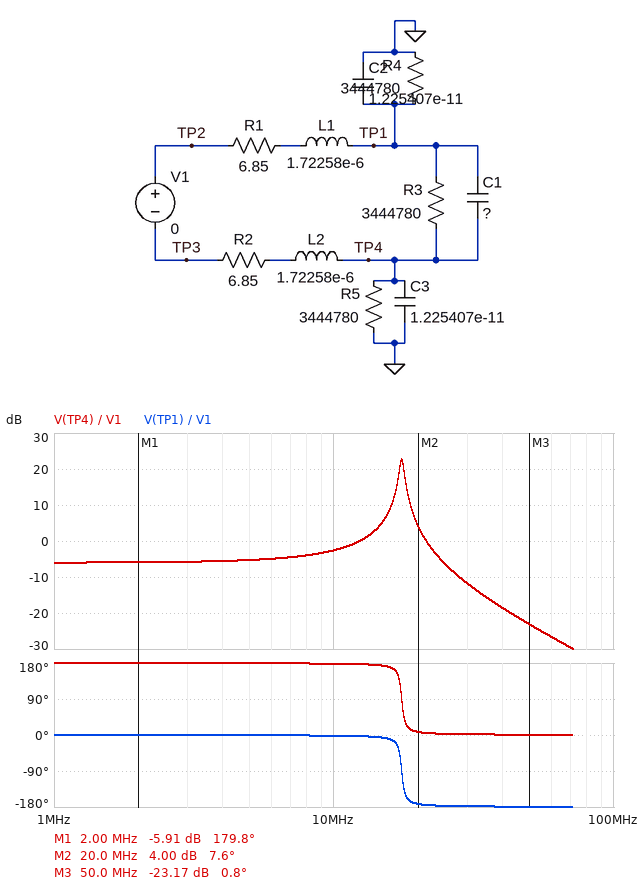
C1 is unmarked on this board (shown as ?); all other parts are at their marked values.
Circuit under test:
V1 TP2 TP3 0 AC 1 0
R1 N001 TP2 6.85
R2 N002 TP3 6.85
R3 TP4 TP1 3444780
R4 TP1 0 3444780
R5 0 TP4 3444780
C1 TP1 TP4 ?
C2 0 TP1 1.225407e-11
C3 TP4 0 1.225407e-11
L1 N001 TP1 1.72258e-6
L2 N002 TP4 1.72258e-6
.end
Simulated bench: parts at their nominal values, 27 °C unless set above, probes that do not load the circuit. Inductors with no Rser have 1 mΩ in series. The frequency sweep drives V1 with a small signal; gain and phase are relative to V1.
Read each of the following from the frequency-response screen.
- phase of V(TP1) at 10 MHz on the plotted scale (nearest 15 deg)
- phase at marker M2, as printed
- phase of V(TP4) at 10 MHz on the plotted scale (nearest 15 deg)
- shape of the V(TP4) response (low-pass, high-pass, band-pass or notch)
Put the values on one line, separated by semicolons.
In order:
0 deg; 7.6 deg; 180 deg; low-pass
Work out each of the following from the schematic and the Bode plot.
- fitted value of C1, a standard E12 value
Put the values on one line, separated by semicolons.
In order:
18 pF
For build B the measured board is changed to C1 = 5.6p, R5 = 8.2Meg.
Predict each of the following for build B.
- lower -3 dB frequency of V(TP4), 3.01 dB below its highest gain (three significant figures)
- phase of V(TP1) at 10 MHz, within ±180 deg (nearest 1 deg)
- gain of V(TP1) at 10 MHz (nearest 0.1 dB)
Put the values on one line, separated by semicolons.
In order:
24.7 MHz; -1 deg; -4.5 dB
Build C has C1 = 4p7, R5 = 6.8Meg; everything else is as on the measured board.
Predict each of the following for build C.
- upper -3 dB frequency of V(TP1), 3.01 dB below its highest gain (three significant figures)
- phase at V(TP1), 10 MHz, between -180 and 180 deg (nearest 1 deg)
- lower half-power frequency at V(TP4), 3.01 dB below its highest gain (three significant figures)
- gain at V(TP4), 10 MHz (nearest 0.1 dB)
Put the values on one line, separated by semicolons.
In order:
26.4 MHz; -1 deg; 25.7 MHz; -4.6 dB
